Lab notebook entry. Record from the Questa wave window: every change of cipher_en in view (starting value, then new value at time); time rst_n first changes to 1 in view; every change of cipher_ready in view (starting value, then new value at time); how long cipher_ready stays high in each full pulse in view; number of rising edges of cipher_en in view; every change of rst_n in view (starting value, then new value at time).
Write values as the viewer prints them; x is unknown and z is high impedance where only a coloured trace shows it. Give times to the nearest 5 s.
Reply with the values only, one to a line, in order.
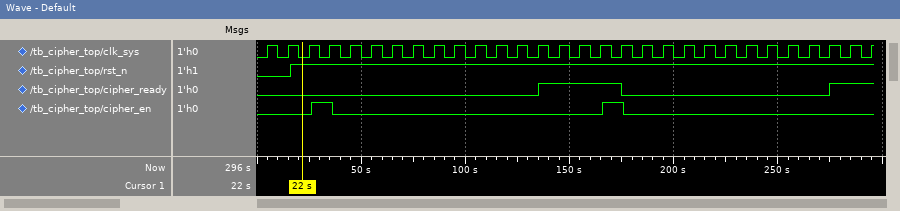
0, 1 at 25 s, 0 at 35 s, 1 at 165 s, 0 at 175 s
15 s
0, 1 at 135 s, 0 at 175 s, 1 at 275 s
40 s
2
0, 1 at 15 s
